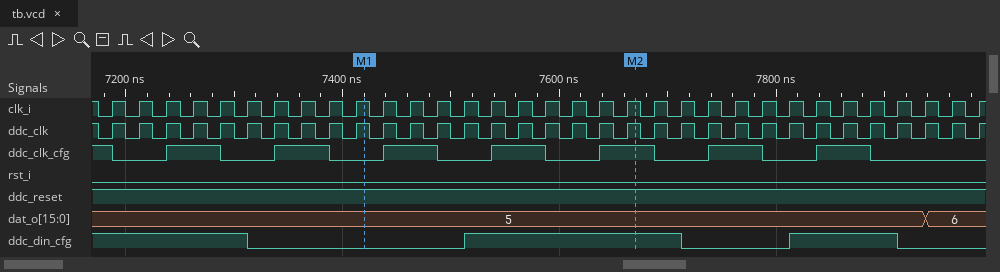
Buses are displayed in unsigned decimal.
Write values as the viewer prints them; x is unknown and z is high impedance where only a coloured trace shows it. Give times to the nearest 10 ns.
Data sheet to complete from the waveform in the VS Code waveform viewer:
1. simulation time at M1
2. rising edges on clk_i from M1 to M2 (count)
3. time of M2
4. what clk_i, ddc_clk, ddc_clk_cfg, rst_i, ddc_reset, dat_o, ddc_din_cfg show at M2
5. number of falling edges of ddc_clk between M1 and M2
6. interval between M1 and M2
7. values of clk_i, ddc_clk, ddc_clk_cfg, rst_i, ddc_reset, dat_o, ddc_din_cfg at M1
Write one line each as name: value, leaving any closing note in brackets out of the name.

simulation time at M1: 7420 ns
rising edges on clk_i from M1 to M2: 10
time of M2: 7670 ns
what clk_i, ddc_clk, ddc_clk_cfg, rst_i, ddc_reset, dat_o, ddc_din_cfg show at M2: clk_i=1, ddc_clk=1, ddc_clk_cfg=1, rst_i=0, ddc_reset=1, dat_o=5, ddc_din_cfg=1
number of falling edges of ddc_clk between M1 and M2: 10
interval between M1 and M2: 250 ns
values of clk_i, ddc_clk, ddc_clk_cfg, rst_i, ddc_reset, dat_o, ddc_din_cfg at M1: clk_i=1, ddc_clk=1, ddc_clk_cfg=0, rst_i=0, ddc_reset=1, dat_o=5, ddc_din_cfg=0
